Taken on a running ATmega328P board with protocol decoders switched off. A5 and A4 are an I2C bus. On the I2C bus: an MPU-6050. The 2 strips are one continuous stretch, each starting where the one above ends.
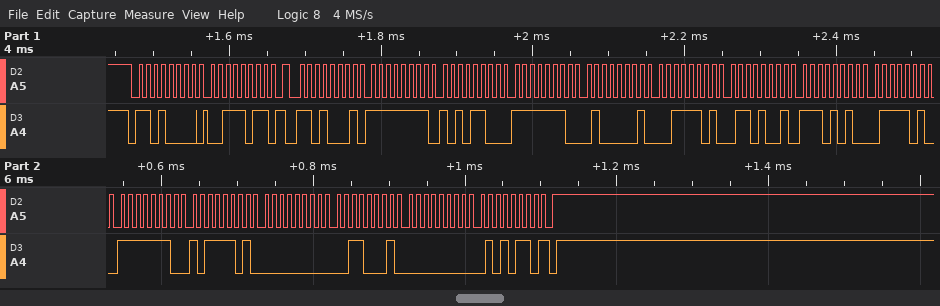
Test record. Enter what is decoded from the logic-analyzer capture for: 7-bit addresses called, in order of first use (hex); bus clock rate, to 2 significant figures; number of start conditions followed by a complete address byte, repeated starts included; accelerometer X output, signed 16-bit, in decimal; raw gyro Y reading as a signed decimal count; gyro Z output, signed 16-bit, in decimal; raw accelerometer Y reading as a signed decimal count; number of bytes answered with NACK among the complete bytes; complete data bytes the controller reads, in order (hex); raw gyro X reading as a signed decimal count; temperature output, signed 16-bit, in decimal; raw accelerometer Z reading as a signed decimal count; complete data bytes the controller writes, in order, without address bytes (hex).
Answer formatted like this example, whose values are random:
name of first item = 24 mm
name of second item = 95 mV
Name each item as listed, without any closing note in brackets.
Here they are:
7-bit addresses called, in order of first use = 0x68
bus clock rate, to 2 significant figures = 100 kHz
number of start conditions followed by a complete address byte, repeated starts included = 2
accelerometer X output, signed 16-bit, in decimal = -84
raw gyro Y reading as a signed decimal count = 49
gyro Z output, signed 16-bit, in decimal = 86
raw accelerometer Y reading as a signed decimal count = -447
number of bytes answered with NACK among the complete bytes = 1
complete data bytes the controller reads, in order = FF AC FE 41 3D 69 EA 7A FE BD 00 31 00 56
raw gyro X reading as a signed decimal count = -323
temperature output, signed 16-bit, in decimal = -5510
raw accelerometer Z reading as a signed decimal count = 15721
complete data bytes the controller writes, in order, without address bytes = 3B
